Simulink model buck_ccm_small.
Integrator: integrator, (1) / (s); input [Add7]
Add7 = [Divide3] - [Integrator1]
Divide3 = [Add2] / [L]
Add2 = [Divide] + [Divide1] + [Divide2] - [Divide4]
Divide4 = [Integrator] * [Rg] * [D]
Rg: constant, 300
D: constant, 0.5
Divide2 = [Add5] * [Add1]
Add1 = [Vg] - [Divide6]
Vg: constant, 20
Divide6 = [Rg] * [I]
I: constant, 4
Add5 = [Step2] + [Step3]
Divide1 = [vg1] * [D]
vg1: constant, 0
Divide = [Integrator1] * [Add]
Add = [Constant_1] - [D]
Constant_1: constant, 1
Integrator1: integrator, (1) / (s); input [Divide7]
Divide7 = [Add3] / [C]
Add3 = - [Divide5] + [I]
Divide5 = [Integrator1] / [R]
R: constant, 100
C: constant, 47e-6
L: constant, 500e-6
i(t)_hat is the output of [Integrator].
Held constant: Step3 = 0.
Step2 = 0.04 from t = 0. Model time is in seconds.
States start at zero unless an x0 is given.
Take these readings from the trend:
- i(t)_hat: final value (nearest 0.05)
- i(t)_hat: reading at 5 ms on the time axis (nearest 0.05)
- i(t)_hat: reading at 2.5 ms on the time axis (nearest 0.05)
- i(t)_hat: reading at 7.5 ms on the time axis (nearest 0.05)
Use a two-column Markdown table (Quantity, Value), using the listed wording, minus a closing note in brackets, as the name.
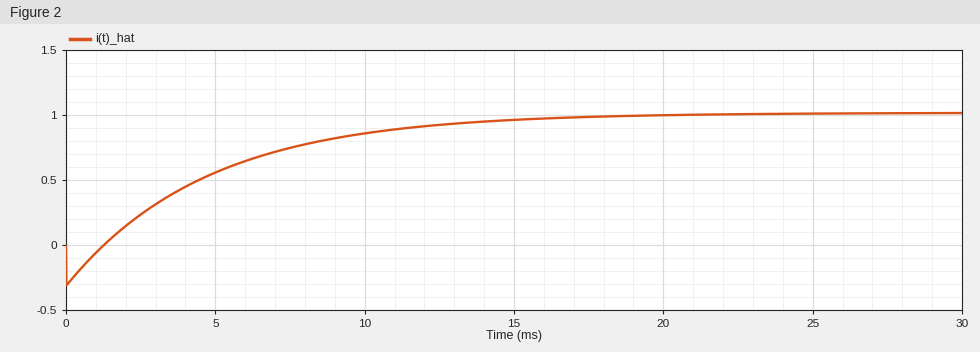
| Quantity | Value |
|---|---|
| i(t)_hat: final value | 1.00 |
| i(t)_hat: reading at 5 ms on the time axis | 0.55 |
| i(t)_hat: reading at 2.5 ms on the time axis | 0.25 |
| i(t)_hat: reading at 7.5 ms on the time axis | 0.75 |
